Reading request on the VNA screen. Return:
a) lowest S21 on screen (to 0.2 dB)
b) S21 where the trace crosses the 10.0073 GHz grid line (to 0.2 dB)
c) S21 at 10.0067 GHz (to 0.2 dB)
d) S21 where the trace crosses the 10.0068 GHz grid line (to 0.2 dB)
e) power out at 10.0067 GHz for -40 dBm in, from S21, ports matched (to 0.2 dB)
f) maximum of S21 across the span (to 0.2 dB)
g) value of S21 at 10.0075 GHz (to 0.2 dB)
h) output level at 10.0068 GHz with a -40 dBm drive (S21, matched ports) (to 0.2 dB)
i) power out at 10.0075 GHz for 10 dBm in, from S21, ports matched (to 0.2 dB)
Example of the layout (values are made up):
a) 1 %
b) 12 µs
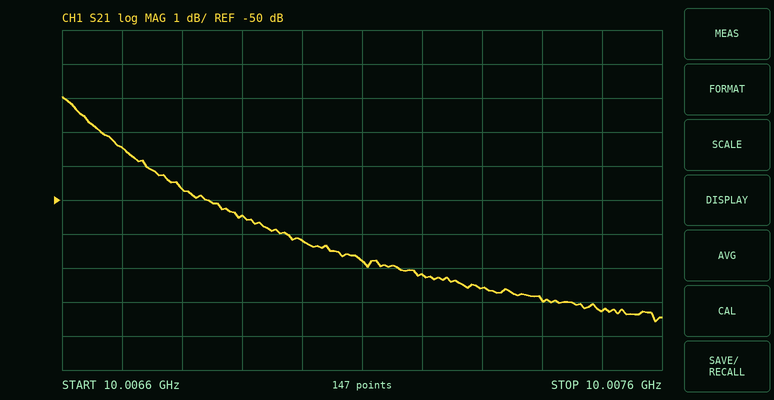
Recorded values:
a) -53.6 dB
b) -52.6 dB
c) -48.4 dB
d) -49.6 dB
e) -88.4 dBm
f) -47.0 dB
g) -53.2 dB
h) -89.6 dBm
i) -43.2 dBm
